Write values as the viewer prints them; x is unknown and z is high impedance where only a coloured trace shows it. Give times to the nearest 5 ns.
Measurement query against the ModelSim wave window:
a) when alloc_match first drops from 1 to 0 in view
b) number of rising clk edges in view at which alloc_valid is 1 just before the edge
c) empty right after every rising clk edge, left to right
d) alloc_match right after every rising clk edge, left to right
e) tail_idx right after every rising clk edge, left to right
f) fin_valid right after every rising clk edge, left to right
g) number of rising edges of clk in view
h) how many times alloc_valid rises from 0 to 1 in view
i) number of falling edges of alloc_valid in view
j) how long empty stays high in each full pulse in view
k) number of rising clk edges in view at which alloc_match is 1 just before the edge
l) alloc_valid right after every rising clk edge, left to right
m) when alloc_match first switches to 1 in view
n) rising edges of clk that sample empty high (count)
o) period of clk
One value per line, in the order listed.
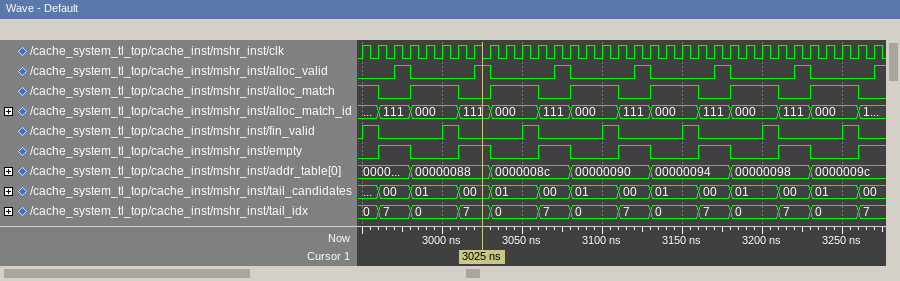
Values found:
2960 ns
6
0 1 1 0 0 0 1 1 0 0 0 1 1 0 0 0 1 1 0 0 0 1 1 0 0 0 1 1 0 0 0 1 1
1 0 0 1 1 1 0 0 1 1 1 0 0 1 1 1 0 0 1 1 1 0 0 1 1 1 0 0 1 1 1 0 0
0, 7, 7, 0, 0, 0, 7, 7, 0, 0, 0, 7, 7, 0, 0, 0, 7, 7, 0, 0, 0, 7, 7, 0, 0, 0, 7, 7, 0, 0, 0, 7, 7
1 0 0 0 0 1 0 0 0 0 1 0 0 0 0 1 0 0 0 0 1 0 0 0 0 1 0 0 0 0 1 0 0
33
7
6
20 ns, 20 ns, 20 ns, 20 ns, 20 ns, 20 ns
20
0 0 1 0 0 0 0 1 0 0 0 0 1 0 0 0 0 1 0 0 0 0 1 0 0 0 0 1 0 0 0 0 1
2980 ns
13
10 ns
